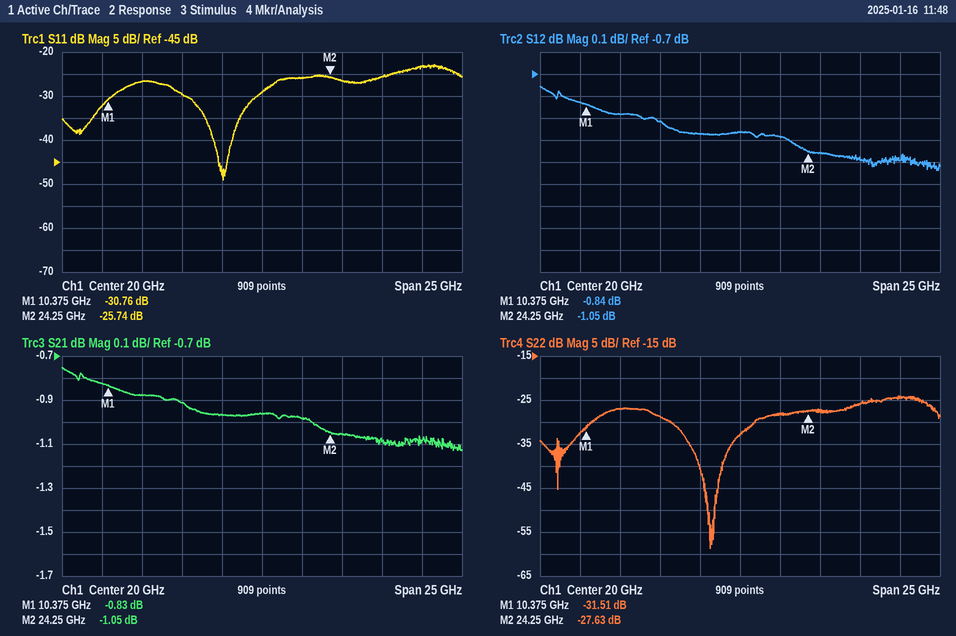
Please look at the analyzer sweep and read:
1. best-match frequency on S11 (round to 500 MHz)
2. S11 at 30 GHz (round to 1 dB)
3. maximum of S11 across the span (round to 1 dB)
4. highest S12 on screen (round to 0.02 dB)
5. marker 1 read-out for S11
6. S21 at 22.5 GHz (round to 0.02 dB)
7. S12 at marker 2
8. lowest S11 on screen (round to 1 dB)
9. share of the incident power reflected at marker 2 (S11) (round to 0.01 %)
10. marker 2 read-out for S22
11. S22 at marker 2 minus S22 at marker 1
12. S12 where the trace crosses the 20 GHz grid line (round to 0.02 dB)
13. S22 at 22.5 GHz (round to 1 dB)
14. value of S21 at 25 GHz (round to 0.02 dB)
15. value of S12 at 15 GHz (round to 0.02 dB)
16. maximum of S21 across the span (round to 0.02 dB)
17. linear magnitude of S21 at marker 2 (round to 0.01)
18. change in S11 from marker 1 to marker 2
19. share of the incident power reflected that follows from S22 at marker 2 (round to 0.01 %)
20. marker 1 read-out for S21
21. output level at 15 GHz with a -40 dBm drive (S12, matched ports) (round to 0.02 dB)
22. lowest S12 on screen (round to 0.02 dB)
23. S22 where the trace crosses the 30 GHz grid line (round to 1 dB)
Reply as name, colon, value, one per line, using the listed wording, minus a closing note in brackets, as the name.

best-match frequency on S11: 17.5 GHz
S11 at 30 GHz: -23 dB
maximum of S11 across the span: -23 dB
highest S12 on screen: -0.76 dB
marker 1 read-out for S11: -30.76 dB
S21 at 22.5 GHz: -0.98 dB
S12 at marker 2: -1.05 dB
lowest S11 on screen: -49 dB
share of the incident power reflected at marker 2 (S11): 0.27 %
marker 2 read-out for S22: -27.63 dB
S22 at marker 2 minus S22 at marker 1: 3.88 dB
S12 where the trace crosses the 20 GHz grid line: -0.96 dB
S22 at 22.5 GHz: -28 dB
value of S21 at 25 GHz: -1.06 dB
value of S12 at 15 GHz: -0.92 dB
maximum of S21 across the span: -0.76 dB
linear magnitude of S21 at marker 2: 0.89
change in S11 from marker 1 to marker 2: 5.02 dB
share of the incident power reflected that follows from S22 at marker 2: 0.17 %
marker 1 read-out for S21: -0.83 dB
output level at 15 GHz with a -40 dBm drive (S12, matched ports): -40.92 dBm
lowest S12 on screen: -1.14 dB
S22 where the trace crosses the 30 GHz grid line: -24 dB
